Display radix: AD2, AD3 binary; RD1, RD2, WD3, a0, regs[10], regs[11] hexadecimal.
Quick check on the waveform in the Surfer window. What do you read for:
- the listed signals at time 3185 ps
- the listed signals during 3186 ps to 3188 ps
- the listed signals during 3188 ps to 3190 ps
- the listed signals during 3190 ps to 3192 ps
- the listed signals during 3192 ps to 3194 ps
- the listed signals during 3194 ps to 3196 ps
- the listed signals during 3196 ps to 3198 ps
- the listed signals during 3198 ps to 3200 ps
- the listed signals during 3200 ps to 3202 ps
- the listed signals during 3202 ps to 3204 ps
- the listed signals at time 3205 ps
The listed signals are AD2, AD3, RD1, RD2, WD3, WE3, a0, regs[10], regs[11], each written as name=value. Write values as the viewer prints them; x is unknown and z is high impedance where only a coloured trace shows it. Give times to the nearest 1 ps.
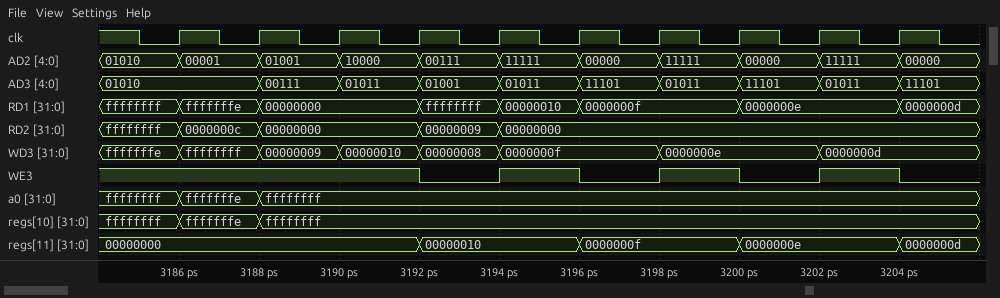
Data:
AD2=01010, AD3=01010, RD1=ffffffff, RD2=ffffffff, WD3=fffffffe, WE3=1, a0=ffffffff, regs[10]=ffffffff, regs[11]=00000000
AD2=00001, AD3=01010, RD1=fffffffe, RD2=0000000c, WD3=ffffffff, WE3=1, a0=fffffffe, regs[10]=fffffffe, regs[11]=00000000
AD2=01001, AD3=00111, RD1=00000000, RD2=00000000, WD3=00000009, WE3=1, a0=ffffffff, regs[10]=ffffffff, regs[11]=00000000
AD2=10000, AD3=01011, RD1=00000000, RD2=00000000, WD3=00000010, WE3=1, a0=ffffffff, regs[10]=ffffffff, regs[11]=00000000
AD2=00111, AD3=01001, RD1=ffffffff, RD2=00000009, WD3=00000008, WE3=0, a0=ffffffff, regs[10]=ffffffff, regs[11]=00000010
AD2=11111, AD3=01011, RD1=00000010, RD2=00000000, WD3=0000000f, WE3=1, a0=ffffffff, regs[10]=ffffffff, regs[11]=00000010
AD2=00000, AD3=11101, RD1=0000000f, RD2=00000000, WD3=0000000f, WE3=0, a0=ffffffff, regs[10]=ffffffff, regs[11]=0000000f
AD2=11111, AD3=01011, RD1=0000000f, RD2=00000000, WD3=0000000e, WE3=1, a0=ffffffff, regs[10]=ffffffff, regs[11]=0000000f
AD2=00000, AD3=11101, RD1=0000000e, RD2=00000000, WD3=0000000e, WE3=0, a0=ffffffff, regs[10]=ffffffff, regs[11]=0000000e
AD2=11111, AD3=01011, RD1=0000000e, RD2=00000000, WD3=0000000d, WE3=1, a0=ffffffff, regs[10]=ffffffff, regs[11]=0000000e
AD2=00000, AD3=11101, RD1=0000000d, RD2=00000000, WD3=0000000d, WE3=0, a0=ffffffff, regs[10]=ffffffff, regs[11]=0000000d
